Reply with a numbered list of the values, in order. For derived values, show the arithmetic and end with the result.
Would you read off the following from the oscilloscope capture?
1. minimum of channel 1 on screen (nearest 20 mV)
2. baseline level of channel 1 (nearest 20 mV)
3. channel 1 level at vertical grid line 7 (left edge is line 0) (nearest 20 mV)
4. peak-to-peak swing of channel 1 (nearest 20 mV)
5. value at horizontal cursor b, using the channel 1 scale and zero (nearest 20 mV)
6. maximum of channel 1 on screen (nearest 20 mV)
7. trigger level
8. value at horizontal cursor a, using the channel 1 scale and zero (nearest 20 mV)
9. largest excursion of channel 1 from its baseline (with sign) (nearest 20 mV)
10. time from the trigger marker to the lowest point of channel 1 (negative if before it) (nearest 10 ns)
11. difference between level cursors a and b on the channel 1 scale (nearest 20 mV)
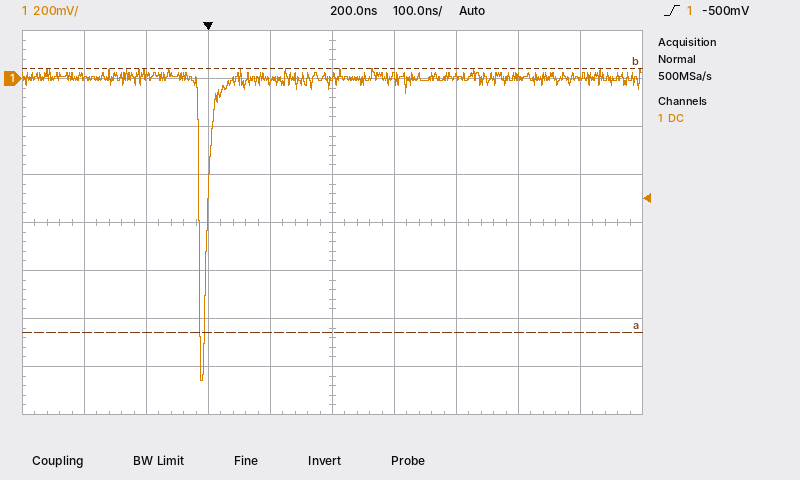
1. -1.26 V
2. 0 mV
3. 0 mV
4. 40 mV − (-1.26 V) = 1.30 V
5. 40 mV
6. 40 mV
7. -500 mV
8. -1.06 V
9. -1.26 V − (0 mV) = -1.26 V
10. -10 ns
11. 1.10 V
